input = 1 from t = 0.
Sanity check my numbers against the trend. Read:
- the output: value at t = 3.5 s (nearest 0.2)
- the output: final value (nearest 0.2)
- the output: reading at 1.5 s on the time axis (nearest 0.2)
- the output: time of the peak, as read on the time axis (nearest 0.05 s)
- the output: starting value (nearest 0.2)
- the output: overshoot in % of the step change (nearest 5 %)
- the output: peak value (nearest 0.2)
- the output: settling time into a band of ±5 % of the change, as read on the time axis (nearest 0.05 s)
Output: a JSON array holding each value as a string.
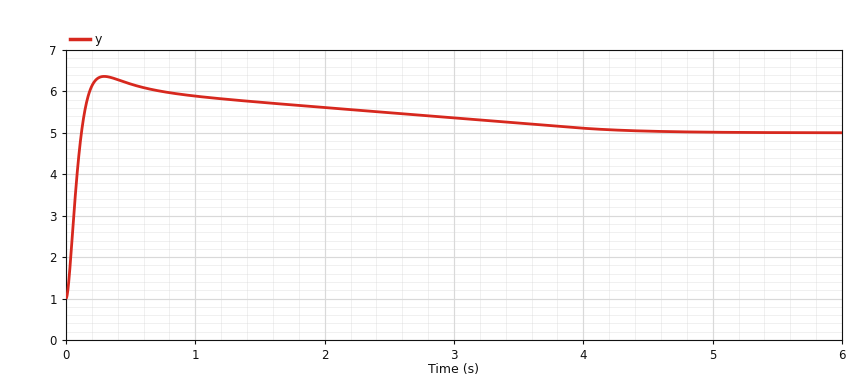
["5.2", "5.0", "5.8", "0.30 s", "1.0", "35 %", "6.4", "3.60 s"]
